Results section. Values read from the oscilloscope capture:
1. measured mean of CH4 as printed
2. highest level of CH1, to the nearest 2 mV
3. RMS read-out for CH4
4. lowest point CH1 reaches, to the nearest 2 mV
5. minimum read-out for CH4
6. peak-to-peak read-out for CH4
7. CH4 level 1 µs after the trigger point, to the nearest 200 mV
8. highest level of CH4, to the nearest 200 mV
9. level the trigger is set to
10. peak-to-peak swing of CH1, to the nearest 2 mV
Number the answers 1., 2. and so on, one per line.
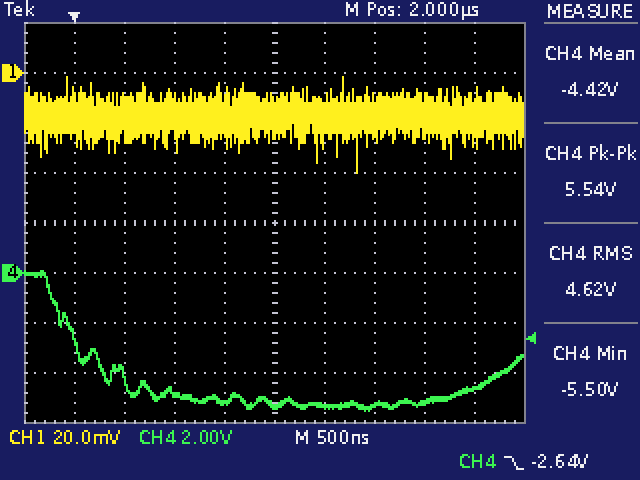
1. -4.42 V
2. -2 mV
3. 4.62 V
4. -40 mV
5. -5.50 V
6. 5.54 V
7. -4.8 V
8. 0.0 V
9. -2.64 V
10. 38 mV
